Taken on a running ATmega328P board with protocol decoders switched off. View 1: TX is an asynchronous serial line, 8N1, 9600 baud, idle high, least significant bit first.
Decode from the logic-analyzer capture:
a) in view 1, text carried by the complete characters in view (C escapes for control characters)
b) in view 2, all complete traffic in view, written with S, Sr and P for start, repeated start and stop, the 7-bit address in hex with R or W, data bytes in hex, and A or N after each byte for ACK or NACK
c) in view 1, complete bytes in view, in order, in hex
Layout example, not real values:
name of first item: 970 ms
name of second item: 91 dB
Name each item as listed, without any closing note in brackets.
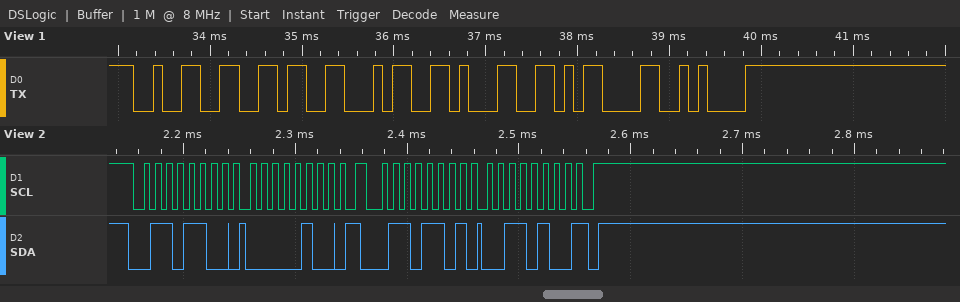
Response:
in view 1, text carried by the complete characters in view: "2641\r\n"
in view 2, all complete traffic in view, written with S, Sr and P for start, repeated start and stop, the 7-bit address in hex with R or W, data bytes in hex, and A or N after each byte for ACK or NACK: S 36W A 04 A Sr 36R A 34 N P
in view 1, complete bytes in view, in order, in hex: 32 36 34 31 0D 0A
